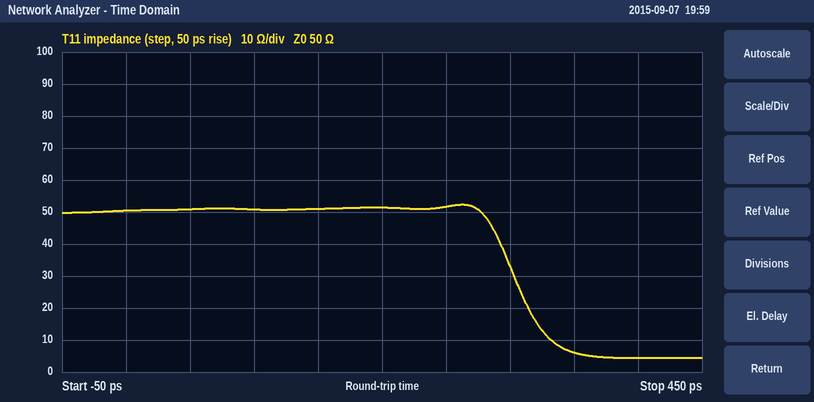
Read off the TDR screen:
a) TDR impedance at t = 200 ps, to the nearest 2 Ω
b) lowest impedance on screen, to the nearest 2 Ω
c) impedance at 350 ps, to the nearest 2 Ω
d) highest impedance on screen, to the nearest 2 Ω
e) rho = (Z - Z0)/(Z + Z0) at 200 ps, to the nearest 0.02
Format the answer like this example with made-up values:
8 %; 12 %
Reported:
52 Ω; 4 Ω; 6 Ω; 52 Ω; +0.02
